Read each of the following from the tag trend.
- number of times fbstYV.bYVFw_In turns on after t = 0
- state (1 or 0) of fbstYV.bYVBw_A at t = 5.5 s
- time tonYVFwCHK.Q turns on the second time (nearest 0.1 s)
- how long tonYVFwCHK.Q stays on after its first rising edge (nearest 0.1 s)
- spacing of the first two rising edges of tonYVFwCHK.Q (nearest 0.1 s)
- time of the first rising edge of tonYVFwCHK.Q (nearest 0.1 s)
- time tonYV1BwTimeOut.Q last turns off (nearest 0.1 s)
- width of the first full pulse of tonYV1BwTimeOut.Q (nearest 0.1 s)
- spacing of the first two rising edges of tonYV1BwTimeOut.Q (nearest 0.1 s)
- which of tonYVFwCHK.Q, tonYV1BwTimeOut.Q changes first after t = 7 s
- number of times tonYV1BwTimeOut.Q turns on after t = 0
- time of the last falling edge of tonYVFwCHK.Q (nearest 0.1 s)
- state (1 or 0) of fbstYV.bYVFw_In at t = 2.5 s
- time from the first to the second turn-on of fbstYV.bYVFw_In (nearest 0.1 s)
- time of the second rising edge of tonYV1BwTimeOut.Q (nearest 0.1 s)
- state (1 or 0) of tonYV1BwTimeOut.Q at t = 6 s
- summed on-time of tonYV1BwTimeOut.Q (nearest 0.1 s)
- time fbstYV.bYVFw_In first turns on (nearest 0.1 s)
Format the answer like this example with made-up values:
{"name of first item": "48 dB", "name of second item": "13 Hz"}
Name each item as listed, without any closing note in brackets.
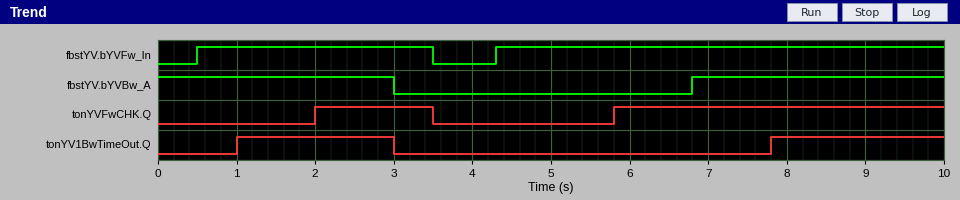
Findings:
{"number of times fbstYV.bYVFw_In turns on after t = 0": "2", "state (1 or 0) of fbstYV.bYVBw_A at t = 5.5 s": "0", "time tonYVFwCHK.Q turns on the second time": "5.8 s", "how long tonYVFwCHK.Q stays on after its first rising edge": "1.5 s", "spacing of the first two rising edges of tonYVFwCHK.Q": "3.8 s", "time of the first rising edge of tonYVFwCHK.Q": "2.0 s", "time tonYV1BwTimeOut.Q last turns off": "3.0 s", "width of the first full pulse of tonYV1BwTimeOut.Q": "2.0 s", "spacing of the first two rising edges of tonYV1BwTimeOut.Q": "6.8 s", "which of tonYVFwCHK.Q, tonYV1BwTimeOut.Q changes first after t = 7 s": "tonYV1BwTimeOut.Q", "number of times tonYV1BwTimeOut.Q turns on after t = 0": "2", "time of the last falling edge of tonYVFwCHK.Q": "3.5 s", "state (1 or 0) of fbstYV.bYVFw_In at t = 2.5 s": "1", "time from the first to the second turn-on of fbstYV.bYVFw_In": "3.8 s", "time of the second rising edge of tonYV1BwTimeOut.Q": "7.8 s", "state (1 or 0) of tonYV1BwTimeOut.Q at t = 6 s": "0", "summed on-time of tonYV1BwTimeOut.Q": "4.2 s", "time fbstYV.bYVFw_In first turns on": "0.5 s"}
